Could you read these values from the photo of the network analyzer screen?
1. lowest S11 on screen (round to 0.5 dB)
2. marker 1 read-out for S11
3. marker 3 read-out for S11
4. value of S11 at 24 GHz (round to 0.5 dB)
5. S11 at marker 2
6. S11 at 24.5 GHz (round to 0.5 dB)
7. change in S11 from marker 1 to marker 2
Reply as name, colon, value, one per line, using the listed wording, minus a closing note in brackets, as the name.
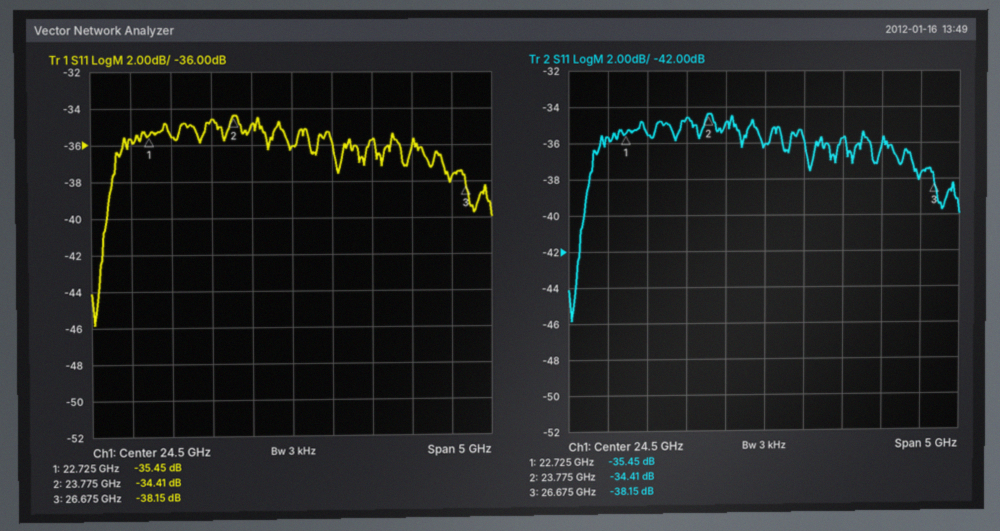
lowest S11 on screen: -46.0 dB
marker 1 read-out for S11: -35.45 dB
marker 3 read-out for S11: -38.15 dB
value of S11 at 24 GHz: -35.0 dB
S11 at marker 2: -34.41 dB
S11 at 24.5 GHz: -36.0 dB
change in S11 from marker 1 to marker 2: 1.04 dB
